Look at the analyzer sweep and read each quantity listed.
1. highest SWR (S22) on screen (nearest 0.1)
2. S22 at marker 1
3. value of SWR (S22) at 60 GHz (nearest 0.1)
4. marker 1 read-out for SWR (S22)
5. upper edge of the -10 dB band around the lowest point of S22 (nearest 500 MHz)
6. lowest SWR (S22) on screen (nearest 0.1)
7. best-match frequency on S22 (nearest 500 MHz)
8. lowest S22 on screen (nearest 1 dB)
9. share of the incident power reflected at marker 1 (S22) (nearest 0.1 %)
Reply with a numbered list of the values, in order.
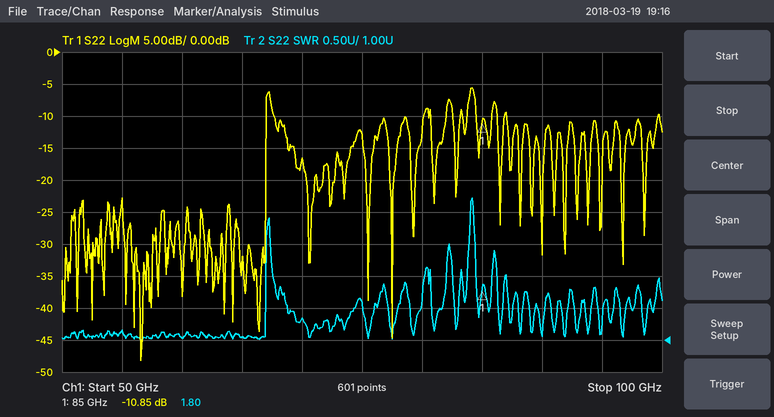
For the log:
1. 3.2
2. -10.85 dB
3. 1.0
4. 1.80
5. 67.0 GHz
6. 1.0
7. 56.5 GHz
8. -48 dB
9. 8.2 %
